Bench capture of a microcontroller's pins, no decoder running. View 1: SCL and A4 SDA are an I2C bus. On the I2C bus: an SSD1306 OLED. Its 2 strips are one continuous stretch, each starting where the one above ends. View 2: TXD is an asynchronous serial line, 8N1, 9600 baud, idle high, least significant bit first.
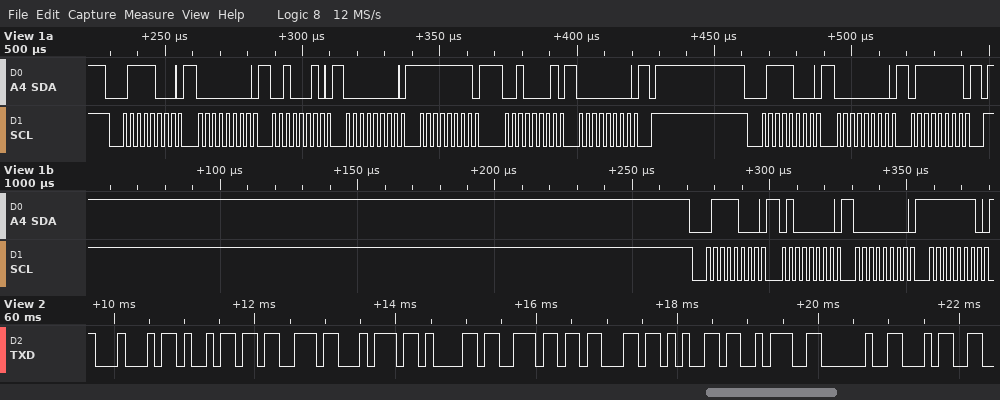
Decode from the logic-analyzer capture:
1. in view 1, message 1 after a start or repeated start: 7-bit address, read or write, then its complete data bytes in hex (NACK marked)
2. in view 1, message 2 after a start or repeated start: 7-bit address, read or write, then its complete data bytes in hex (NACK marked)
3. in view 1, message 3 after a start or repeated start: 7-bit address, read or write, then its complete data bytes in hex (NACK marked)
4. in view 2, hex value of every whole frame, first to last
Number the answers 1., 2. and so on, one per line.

1. 0x3C write: 00 22 00 FF 21 00
2. 0x3C write: 00 7F
3. 0x3C write: 40 00 FE
4. 0x44 0x69 0x73 0x74 0x61 0x6E 0x63 0x65 0x3A 0x20 0x34
